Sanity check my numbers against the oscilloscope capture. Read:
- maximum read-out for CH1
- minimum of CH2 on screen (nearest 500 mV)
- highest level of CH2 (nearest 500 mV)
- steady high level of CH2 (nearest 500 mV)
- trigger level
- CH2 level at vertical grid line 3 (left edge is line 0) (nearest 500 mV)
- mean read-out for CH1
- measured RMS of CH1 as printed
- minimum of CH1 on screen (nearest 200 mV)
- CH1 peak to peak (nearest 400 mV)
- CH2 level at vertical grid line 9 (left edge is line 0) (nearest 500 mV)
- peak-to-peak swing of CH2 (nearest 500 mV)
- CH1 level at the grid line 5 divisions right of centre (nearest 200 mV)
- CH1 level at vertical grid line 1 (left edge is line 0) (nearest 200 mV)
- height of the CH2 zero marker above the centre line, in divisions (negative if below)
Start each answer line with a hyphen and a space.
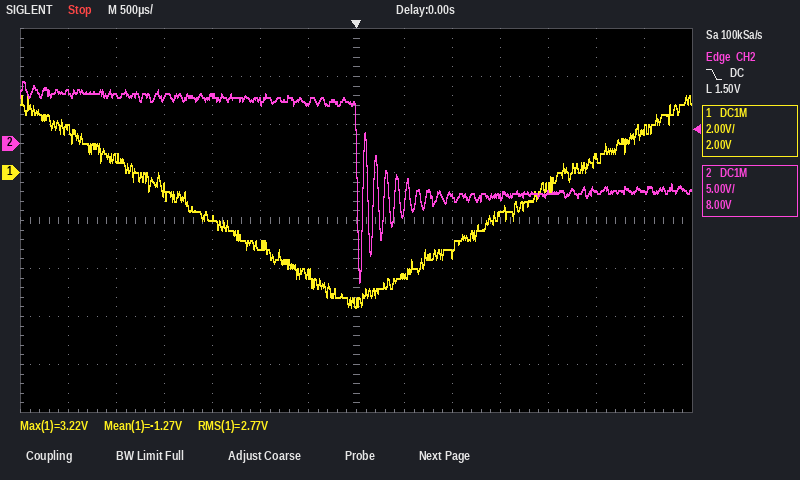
- 3.22 V
- -14.5 V
- 6.5 V
- 5.0 V
- 1.50 V
- 5.0 V
- -1.27 V
- 2.77 V
- -5.6 V
- 8.8 V
- -5.5 V
- 21.0 V
- 600 mV
- 1.8 V
- +1.6 div
